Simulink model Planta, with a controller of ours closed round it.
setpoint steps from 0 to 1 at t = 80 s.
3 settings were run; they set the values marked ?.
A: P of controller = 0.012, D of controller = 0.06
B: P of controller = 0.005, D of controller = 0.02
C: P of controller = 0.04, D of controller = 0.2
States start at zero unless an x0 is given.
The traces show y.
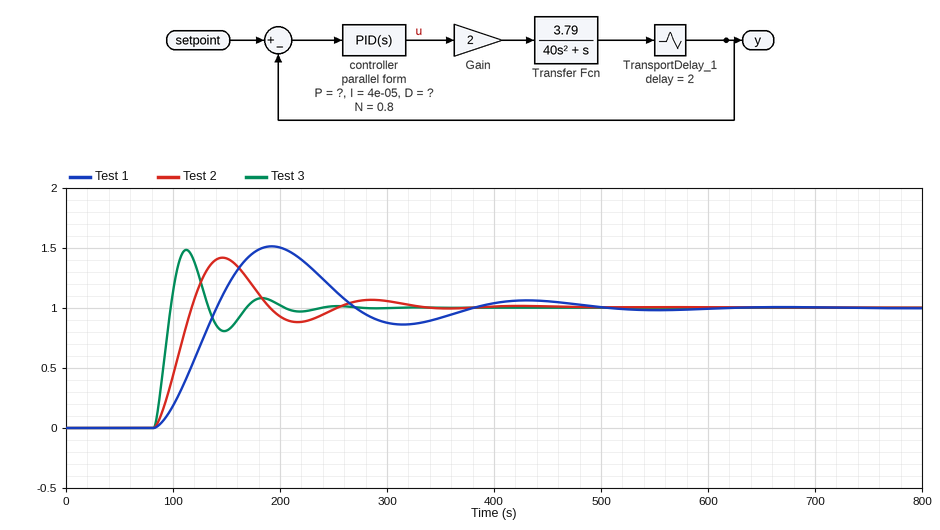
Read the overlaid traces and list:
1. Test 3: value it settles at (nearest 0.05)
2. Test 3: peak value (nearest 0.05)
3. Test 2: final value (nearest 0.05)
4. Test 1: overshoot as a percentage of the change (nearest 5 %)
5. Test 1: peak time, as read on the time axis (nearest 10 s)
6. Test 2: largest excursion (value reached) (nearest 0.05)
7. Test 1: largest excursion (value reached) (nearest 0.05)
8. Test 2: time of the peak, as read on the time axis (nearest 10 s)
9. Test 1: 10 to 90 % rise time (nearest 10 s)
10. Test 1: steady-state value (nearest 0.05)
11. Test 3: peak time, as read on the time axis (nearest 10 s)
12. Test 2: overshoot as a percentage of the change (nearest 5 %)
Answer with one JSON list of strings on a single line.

["1.00", "1.50", "1.00", "50 %", "190 s", "1.40", "1.50", "150 s", "40 s", "1.00", "110 s", "40 %"]
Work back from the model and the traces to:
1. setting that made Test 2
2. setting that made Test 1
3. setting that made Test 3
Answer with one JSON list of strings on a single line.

["A", "B", "C"]
